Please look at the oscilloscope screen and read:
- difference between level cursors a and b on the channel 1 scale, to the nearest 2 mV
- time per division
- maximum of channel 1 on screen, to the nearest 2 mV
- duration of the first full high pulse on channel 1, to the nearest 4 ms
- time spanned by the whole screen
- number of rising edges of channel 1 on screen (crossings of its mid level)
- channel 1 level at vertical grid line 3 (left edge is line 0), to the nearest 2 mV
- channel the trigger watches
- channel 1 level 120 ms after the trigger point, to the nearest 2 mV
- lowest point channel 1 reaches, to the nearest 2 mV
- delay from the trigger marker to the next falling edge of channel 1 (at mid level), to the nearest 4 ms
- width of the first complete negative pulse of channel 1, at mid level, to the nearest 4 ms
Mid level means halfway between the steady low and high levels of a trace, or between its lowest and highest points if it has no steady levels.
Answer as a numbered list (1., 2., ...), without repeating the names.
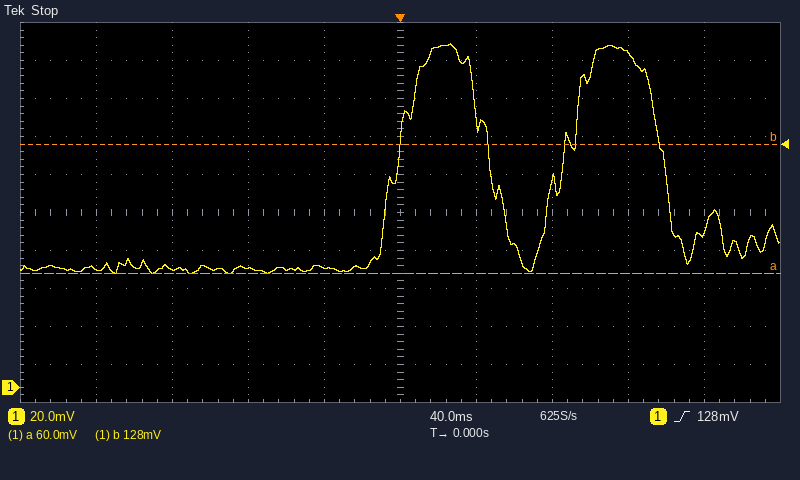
1. 68 mV
2. 40 ms
3. 180 mV
4. 48 ms
5. 400 ms
6. 2
7. 62 mV
8. channel 1
9. 176 mV
10. 60 mV
11. 48 ms
12. 40 ms
